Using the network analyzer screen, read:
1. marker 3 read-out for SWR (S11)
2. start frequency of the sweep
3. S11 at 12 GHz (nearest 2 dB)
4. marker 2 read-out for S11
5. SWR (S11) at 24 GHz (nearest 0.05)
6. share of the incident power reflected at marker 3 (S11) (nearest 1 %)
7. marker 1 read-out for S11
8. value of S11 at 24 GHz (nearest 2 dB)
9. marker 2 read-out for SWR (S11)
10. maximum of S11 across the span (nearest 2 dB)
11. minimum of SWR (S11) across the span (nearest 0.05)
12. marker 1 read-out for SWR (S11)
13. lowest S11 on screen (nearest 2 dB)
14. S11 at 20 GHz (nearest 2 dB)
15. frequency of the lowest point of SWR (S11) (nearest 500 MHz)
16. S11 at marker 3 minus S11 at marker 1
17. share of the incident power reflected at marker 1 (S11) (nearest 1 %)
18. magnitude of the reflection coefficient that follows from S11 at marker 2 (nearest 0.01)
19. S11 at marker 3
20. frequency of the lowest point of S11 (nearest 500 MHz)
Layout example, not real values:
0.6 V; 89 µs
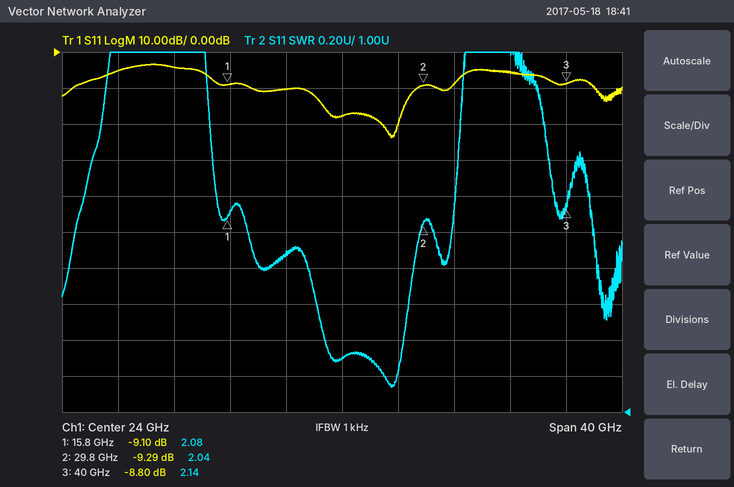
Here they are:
2.14; 4 GHz; -4 dB; -9.29 dB; 1.30; 13 %; -9.10 dB; -18 dB; 2.04; -4 dB; 1.15; 2.08; -24 dB; -10 dB; 27.5 GHz; 0.30 dB; 12 %; 0.34; -8.80 dB; 27.5 GHz
